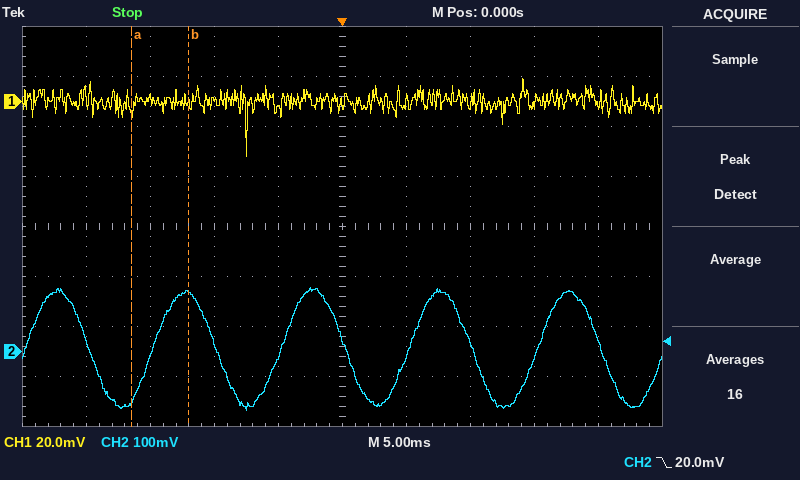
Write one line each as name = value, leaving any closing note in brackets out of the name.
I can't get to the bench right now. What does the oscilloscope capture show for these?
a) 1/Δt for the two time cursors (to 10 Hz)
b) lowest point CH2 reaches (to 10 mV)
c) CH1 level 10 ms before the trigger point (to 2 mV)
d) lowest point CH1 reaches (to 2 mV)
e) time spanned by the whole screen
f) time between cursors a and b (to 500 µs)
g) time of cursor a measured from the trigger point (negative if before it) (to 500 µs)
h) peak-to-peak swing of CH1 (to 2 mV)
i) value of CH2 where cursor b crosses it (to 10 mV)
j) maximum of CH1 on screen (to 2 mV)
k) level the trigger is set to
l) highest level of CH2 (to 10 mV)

1/Δt for the two time cursors = 220 Hz
lowest point CH2 reaches = -120 mV
CH1 level 10 ms before the trigger point = 0 mV
lowest point CH1 reaches = -22 mV
time spanned by the whole screen = 50 ms
time between cursors a and b = 4.5 ms
time of cursor a measured from the trigger point (negative if before it) = -16.5 ms
peak-to-peak swing of CH1 = 32 mV
value of CH2 where cursor b crosses it = 120 mV
maximum of CH1 on screen = 10 mV
level the trigger is set to = 20.0 mV
highest level of CH2 = 130 mV
